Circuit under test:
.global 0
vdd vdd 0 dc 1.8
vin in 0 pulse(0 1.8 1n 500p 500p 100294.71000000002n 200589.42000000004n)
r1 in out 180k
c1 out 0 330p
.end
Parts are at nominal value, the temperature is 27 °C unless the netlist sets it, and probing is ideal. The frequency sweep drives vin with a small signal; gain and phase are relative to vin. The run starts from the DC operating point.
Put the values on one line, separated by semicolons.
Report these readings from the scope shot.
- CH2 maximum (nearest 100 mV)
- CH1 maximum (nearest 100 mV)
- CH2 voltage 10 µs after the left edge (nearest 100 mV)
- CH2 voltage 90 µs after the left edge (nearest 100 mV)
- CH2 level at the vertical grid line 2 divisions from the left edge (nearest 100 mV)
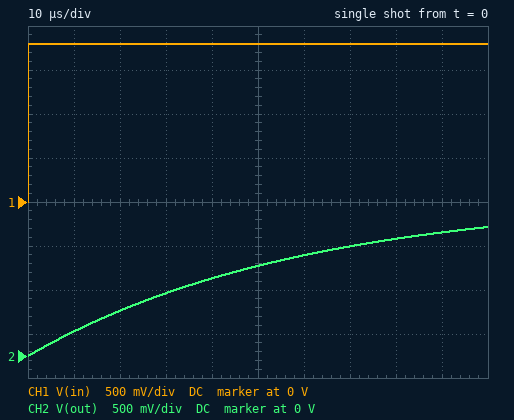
1.5 V; 1.8 V; 300 mV; 1.4 V; 500 mV
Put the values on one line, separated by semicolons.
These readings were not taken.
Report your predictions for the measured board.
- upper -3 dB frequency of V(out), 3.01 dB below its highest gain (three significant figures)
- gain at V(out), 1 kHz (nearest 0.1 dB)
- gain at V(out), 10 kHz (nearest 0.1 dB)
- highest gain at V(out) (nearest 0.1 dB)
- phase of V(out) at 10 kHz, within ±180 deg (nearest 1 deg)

2.68 kHz; -0.6 dB; -11.7 dB; 0 dB; -75 deg
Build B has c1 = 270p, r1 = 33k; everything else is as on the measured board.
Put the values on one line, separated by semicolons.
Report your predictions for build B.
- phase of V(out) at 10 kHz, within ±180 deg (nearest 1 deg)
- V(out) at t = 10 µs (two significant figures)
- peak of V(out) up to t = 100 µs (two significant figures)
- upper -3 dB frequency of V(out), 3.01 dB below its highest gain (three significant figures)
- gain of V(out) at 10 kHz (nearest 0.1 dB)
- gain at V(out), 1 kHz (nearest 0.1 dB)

-29 deg; 1.2 V; 1.8 V; 17.9 kHz; -1.2 dB; 0 dB
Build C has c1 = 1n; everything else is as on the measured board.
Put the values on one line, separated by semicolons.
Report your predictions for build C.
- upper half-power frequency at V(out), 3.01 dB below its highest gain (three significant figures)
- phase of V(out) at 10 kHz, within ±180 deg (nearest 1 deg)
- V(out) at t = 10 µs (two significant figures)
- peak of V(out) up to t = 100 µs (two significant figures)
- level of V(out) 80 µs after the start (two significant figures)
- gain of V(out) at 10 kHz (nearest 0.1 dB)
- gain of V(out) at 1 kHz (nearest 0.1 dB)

884 Hz; -85 deg; 97 mV; 770 mV; 650 mV; -21.1 dB; -3.6 dB
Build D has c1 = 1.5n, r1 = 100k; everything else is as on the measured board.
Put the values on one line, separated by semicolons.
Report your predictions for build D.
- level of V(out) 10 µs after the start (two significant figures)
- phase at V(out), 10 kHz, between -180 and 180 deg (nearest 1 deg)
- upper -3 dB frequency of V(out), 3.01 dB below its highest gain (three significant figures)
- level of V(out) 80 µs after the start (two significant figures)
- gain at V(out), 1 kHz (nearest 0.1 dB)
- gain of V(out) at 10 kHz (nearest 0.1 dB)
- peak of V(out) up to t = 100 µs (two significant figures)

120 mV; -84 deg; 1.06 kHz; 740 mV; -2.8 dB; -19.5 dB; 880 mV
